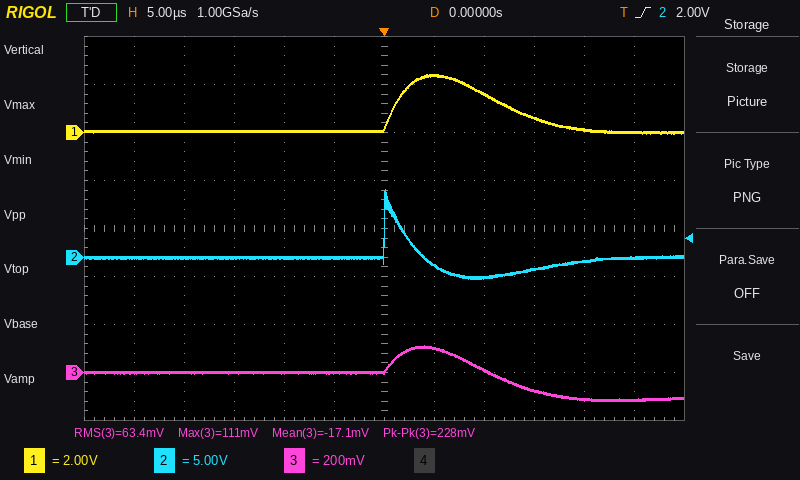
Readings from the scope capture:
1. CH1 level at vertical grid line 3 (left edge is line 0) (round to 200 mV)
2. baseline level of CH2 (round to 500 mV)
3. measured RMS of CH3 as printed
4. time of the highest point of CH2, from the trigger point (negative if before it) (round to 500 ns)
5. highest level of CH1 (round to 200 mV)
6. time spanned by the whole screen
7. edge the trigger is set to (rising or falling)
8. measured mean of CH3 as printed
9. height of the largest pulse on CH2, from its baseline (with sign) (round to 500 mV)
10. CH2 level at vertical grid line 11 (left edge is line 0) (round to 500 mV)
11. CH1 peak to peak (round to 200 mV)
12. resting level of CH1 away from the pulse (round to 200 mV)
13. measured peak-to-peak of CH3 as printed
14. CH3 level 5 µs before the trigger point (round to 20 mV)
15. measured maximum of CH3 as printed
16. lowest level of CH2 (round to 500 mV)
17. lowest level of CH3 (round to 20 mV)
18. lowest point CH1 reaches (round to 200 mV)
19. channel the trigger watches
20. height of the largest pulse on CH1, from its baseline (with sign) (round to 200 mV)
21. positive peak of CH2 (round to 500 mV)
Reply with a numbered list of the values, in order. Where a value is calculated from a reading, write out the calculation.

1. 0.0 V
2. 0.0 V
3. 63.4 mV
4. 0.0 µs
5. 2.4 V
6. 60 µs
7. rising
8. -17.1 mV
9. 7.0 V − (0.0 V) = +7.0 V
10. 0.0 V
11. 2.4 V − (0.0 V) = 2.4 V
12. 0.0 V
13. 228 mV
14. 0 mV
15. 111 mV
16. -2.0 V
17. -120 mV
18. 0.0 V
19. CH2
20. 2.4 V − (0.0 V) = +2.4 V
21. 7.0 V
